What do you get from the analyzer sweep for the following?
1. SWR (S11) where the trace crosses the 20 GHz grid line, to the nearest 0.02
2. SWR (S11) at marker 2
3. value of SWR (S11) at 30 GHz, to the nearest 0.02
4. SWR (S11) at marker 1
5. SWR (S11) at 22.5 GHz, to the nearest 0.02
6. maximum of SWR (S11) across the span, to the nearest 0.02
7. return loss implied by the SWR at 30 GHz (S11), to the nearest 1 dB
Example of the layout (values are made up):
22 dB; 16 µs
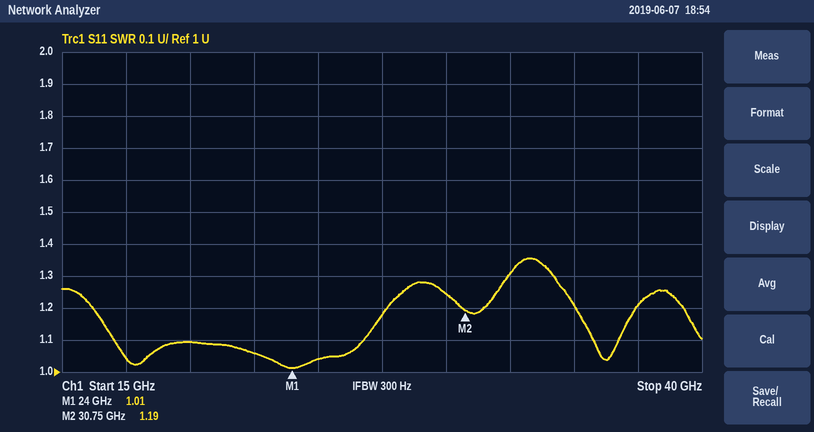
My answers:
1.10; 1.19; 1.24; 1.01; 1.06; 1.36; 19 dB
